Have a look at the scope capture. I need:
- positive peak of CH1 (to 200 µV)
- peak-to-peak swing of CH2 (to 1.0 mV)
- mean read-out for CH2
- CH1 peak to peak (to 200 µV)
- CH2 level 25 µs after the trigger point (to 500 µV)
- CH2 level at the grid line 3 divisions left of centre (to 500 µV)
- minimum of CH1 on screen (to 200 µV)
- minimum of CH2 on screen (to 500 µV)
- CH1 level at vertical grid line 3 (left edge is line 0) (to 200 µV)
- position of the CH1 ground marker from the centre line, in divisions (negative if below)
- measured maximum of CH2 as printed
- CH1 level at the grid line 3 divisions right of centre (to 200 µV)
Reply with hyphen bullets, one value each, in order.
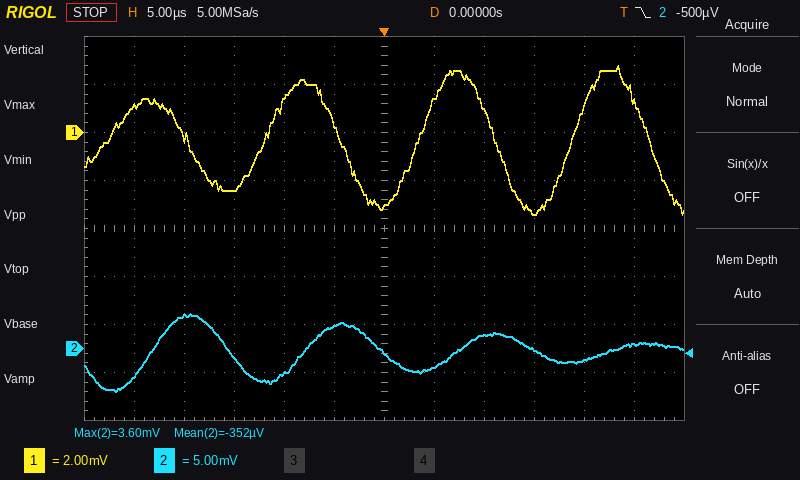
- 2.8 mV
- 8.0 mV
- -352 µV
- 6.2 mV
- 500 µV
- -1.0 mV
- -3.4 mV
- -4.5 mV
- -2.4 mV
- +2.0 div
- 3.60 mV
- -3.4 mV
